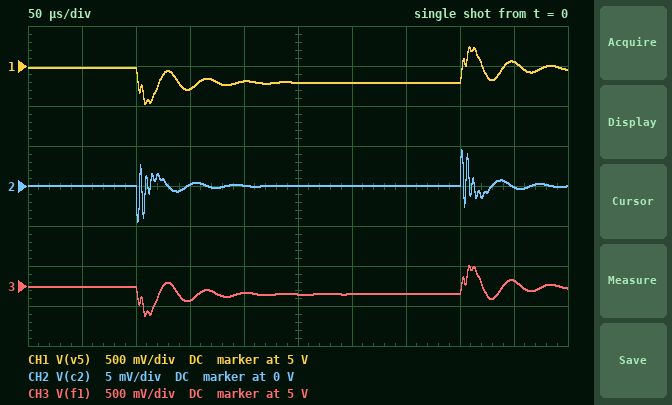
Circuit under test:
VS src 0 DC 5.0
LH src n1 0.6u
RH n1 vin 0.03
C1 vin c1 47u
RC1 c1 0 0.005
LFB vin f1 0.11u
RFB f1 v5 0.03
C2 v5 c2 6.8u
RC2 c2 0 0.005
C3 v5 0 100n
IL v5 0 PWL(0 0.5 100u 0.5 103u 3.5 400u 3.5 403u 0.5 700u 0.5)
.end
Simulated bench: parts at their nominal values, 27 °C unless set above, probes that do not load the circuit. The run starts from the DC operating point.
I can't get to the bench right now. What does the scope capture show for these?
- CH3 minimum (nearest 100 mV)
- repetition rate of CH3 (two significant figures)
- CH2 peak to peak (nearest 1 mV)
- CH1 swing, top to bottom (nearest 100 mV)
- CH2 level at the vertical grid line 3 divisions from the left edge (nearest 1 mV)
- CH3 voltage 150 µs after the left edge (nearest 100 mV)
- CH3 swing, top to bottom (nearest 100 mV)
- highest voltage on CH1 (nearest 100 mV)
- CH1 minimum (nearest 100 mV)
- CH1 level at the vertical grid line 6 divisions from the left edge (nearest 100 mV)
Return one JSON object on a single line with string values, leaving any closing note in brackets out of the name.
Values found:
{"CH3 minimum": "4.6 V", "repetition rate of CH3": "25 kHz", "CH2 peak to peak": "9 mV", "CH1 swing, top to bottom": "700 mV", "CH2 level at the vertical grid line 3 divisions from the left edge": "0 V", "CH3 voltage 150 µs after the left edge": "4.8 V", "CH3 swing, top to bottom": "600 mV", "highest voltage on CH1": "5.2 V", "CH1 minimum": "4.5 V", "CH1 level at the vertical grid line 6 divisions from the left edge": "4.8 V"}
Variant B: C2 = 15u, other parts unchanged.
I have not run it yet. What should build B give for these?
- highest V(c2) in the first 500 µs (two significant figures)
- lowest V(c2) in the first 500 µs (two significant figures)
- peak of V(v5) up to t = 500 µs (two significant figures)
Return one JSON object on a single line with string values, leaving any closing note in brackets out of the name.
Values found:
{"highest V(c2) in the first 500 µs": "7.1 mV", "lowest V(c2) in the first 500 µs": "-7.1 mV", "peak of V(v5) up to t = 500 µs": "5.2 V"}
